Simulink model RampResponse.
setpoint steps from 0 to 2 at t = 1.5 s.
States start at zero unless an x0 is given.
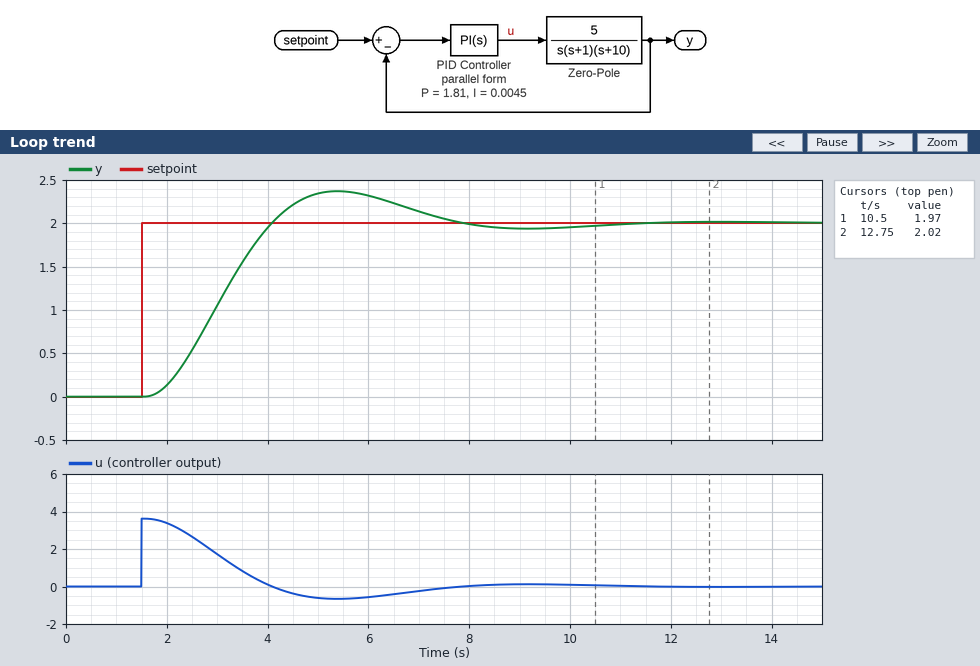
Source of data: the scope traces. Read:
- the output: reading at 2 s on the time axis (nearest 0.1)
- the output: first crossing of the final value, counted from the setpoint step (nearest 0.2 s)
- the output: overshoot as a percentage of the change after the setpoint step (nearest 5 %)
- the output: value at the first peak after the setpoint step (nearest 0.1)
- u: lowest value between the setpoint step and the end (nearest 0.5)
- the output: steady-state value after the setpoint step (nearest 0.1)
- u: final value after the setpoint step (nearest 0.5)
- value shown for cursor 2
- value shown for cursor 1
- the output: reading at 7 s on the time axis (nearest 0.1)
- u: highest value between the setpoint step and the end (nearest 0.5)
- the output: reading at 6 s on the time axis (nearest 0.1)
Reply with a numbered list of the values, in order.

1. 0.1
2. 2.6 s
3. 20 %
4. 2.4
5. -0.5
6. 2.0
7. 0.0
8. 2.02
9. 1.97
10. 2.1
11. 3.5
12. 2.3
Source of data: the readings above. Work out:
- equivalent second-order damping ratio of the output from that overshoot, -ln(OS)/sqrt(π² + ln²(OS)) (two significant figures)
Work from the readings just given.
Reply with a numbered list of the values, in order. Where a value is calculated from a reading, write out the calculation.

1. ln(0.2) = -1.609; 1.609 / sqrt(9.870 + 2.590) = 0.46
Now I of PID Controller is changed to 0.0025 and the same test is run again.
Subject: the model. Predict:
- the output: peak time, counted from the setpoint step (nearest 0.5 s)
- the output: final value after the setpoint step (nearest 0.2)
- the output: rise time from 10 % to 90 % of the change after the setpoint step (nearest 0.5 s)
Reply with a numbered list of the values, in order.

1. 4.0 s
2. 2.0
3. 1.5 s
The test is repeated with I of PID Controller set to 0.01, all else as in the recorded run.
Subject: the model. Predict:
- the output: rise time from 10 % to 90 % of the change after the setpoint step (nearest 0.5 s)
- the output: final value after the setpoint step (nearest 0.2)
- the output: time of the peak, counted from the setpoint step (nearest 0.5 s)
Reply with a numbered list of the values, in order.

1. 1.5 s
2. 2.0
3. 4.0 s
